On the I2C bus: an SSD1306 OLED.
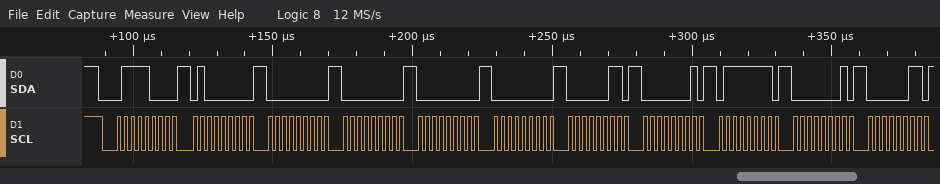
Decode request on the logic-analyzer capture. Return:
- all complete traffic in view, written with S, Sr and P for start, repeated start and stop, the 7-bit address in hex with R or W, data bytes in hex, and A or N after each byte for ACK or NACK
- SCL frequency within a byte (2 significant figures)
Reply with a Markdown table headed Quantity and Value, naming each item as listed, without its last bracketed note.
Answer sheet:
| Quantity | Value |
|---|---|
| all complete traffic in view, written with S, Sr and P for start, repeated start and stop, the 7-bit address in hex with R or W, data bytes in hex, and A or N after each byte for ACK or NACK | S 3CW A 40 A 00 A 00 A 00 A 00 A 03 A 01 A 7F A 01 A 03 A |
| SCL frequency within a byte | 400 kHz |
